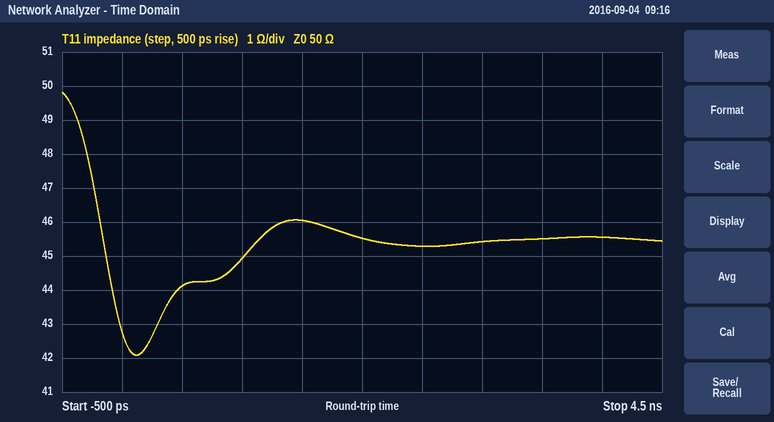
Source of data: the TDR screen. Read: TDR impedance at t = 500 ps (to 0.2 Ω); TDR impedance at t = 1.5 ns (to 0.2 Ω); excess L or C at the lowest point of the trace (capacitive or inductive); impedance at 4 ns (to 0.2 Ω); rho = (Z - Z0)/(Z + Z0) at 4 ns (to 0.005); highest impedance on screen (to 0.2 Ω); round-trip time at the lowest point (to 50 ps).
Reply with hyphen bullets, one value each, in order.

- 44.2 Ω
- 46.0 Ω
- capacitive
- 45.6 Ω
- -0.045
- 49.8 Ω
- 100 ps
